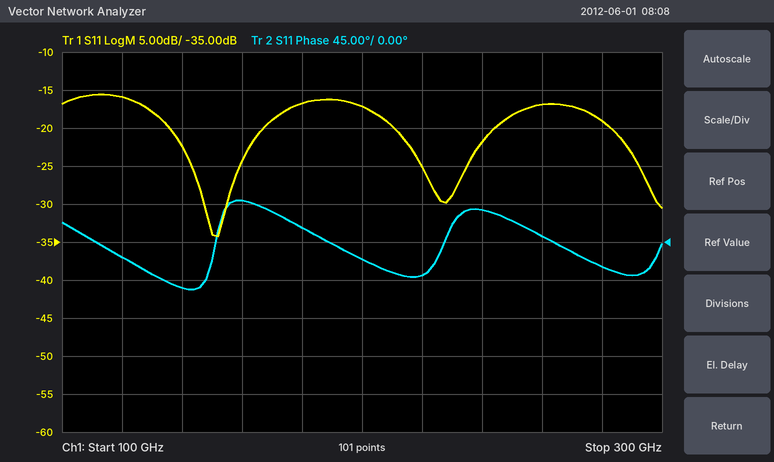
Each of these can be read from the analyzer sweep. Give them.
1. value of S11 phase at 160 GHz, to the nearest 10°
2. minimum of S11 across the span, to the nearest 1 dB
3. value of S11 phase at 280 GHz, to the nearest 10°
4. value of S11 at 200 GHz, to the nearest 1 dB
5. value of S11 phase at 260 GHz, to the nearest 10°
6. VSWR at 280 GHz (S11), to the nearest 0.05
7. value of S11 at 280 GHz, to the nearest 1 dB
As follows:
50°
-34 dB
-30°
-17 dB
10°
1.25
-19 dB
